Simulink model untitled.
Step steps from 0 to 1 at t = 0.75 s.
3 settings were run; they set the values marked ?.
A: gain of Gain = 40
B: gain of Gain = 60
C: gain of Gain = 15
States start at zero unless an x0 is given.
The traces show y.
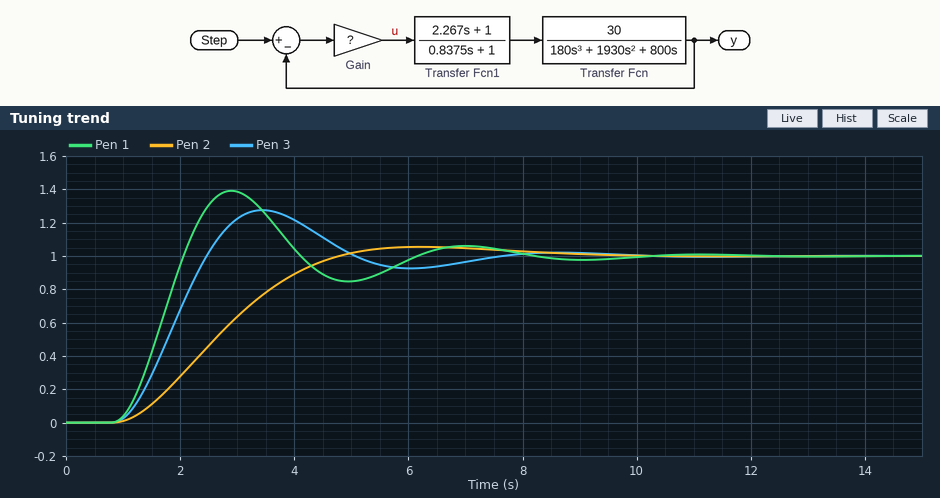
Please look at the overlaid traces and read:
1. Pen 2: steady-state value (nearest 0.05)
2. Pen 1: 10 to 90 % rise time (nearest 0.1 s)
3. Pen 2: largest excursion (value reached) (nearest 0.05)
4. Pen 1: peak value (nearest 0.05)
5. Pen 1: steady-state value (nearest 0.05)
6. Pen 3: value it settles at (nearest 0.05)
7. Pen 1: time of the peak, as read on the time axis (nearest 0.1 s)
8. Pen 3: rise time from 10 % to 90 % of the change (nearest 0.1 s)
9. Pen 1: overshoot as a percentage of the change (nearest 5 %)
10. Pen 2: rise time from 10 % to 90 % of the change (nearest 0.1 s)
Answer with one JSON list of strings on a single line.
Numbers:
["1.00", "0.8 s", "1.05", "1.40", "1.00", "1.00", "2.9 s", "1.1 s", "40 %", "2.6 s"]
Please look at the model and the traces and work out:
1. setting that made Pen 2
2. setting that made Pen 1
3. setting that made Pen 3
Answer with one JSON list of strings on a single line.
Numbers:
["C", "B", "A"]
